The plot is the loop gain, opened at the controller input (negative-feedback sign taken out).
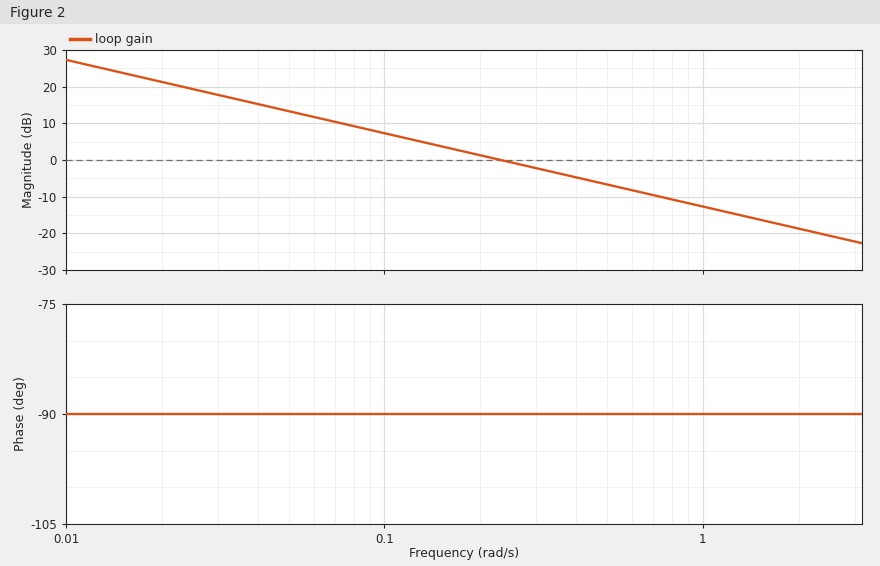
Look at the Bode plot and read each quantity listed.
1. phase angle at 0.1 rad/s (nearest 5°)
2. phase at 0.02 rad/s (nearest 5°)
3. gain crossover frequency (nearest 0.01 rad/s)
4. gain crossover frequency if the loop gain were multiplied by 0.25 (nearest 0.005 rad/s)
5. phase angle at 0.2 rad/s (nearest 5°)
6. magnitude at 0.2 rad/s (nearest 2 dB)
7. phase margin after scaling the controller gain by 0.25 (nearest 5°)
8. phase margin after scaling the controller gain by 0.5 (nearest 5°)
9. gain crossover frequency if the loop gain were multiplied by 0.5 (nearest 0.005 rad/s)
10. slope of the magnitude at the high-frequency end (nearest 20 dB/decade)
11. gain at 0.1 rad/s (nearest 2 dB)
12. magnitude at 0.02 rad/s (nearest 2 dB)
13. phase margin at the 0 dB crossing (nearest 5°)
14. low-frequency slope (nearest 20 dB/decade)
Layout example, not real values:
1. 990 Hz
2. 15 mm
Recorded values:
1. -90°
2. -90°
3. 0.23 rad/s
4. 0.060 rad/s
5. -90°
6. 2 dB
7. 90°
8. 90°
9. 0.115 rad/s
10. -20 dB/decade
11. 8 dB
12. 22 dB
13. 90°
14. -20 dB/decade
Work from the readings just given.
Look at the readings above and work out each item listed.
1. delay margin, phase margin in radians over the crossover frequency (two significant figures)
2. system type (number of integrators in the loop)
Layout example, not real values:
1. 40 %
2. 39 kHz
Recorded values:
1. 6.8 s
2. 1
